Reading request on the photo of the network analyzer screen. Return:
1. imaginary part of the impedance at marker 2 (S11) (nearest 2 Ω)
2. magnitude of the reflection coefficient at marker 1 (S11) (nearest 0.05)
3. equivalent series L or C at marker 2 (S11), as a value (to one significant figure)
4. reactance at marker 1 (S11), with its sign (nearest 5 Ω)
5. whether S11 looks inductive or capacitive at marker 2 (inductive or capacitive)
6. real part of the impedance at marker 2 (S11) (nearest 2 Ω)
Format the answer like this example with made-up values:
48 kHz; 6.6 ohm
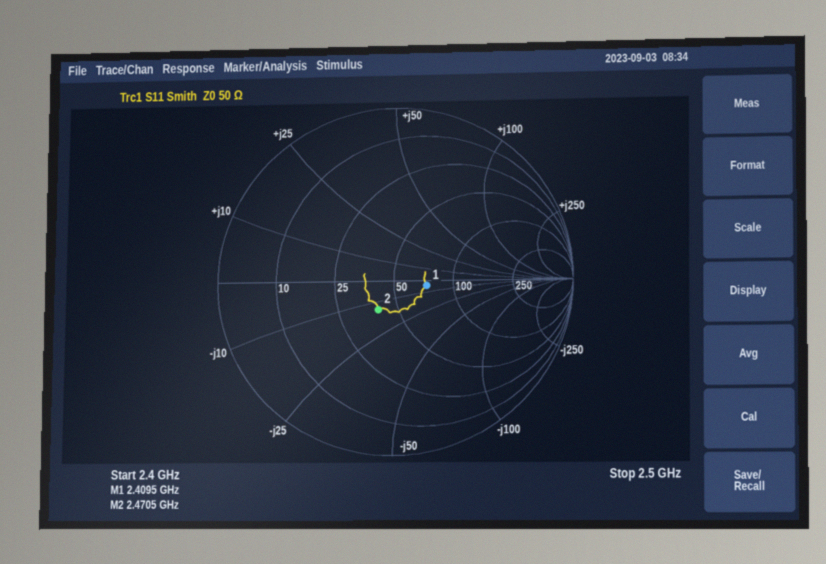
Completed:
-14 Ω; 0.20; 5 pF; -5 Ω; capacitive; 40 Ω
